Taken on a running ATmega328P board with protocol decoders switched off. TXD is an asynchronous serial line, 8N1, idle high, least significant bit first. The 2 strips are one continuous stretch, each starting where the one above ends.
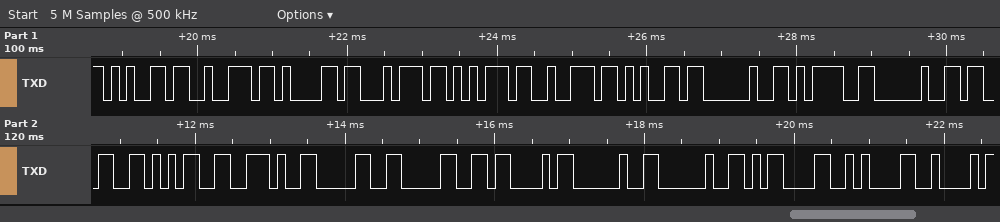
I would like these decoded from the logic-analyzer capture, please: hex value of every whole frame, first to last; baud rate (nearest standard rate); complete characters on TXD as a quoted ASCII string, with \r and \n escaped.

65 72 61 74 75 72 65 20 3D 20 33 35 2E 30 30 43 20 20 0D 0A 42
9600 baud
"erature = 35.00C  \r\nB"
